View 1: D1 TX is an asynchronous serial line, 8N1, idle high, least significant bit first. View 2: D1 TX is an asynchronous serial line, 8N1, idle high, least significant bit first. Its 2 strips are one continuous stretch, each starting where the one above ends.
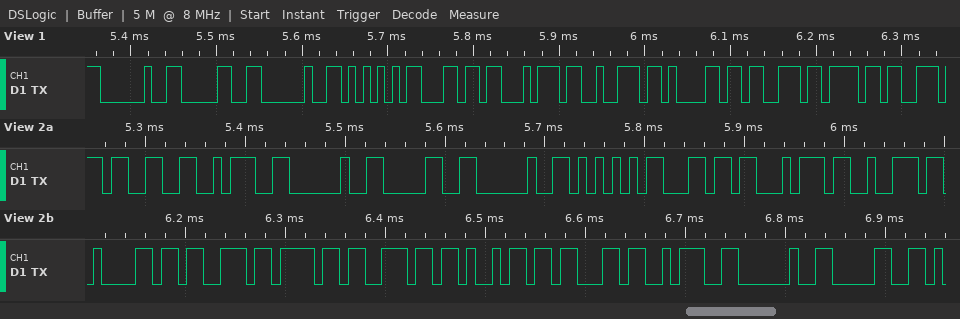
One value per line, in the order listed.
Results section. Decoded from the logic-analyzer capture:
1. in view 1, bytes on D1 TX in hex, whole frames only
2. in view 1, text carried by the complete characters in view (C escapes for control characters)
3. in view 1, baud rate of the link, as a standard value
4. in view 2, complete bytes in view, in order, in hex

0x20 0x30 0x20 0x55 0x6C 0x74 0x72 0x61 0x73 0x6F
" 0 Ultraso"
115200 baud
33 3A 20 30 20 55 6C 74 72 61 73 6F 6E 69 63 3A 20 30
